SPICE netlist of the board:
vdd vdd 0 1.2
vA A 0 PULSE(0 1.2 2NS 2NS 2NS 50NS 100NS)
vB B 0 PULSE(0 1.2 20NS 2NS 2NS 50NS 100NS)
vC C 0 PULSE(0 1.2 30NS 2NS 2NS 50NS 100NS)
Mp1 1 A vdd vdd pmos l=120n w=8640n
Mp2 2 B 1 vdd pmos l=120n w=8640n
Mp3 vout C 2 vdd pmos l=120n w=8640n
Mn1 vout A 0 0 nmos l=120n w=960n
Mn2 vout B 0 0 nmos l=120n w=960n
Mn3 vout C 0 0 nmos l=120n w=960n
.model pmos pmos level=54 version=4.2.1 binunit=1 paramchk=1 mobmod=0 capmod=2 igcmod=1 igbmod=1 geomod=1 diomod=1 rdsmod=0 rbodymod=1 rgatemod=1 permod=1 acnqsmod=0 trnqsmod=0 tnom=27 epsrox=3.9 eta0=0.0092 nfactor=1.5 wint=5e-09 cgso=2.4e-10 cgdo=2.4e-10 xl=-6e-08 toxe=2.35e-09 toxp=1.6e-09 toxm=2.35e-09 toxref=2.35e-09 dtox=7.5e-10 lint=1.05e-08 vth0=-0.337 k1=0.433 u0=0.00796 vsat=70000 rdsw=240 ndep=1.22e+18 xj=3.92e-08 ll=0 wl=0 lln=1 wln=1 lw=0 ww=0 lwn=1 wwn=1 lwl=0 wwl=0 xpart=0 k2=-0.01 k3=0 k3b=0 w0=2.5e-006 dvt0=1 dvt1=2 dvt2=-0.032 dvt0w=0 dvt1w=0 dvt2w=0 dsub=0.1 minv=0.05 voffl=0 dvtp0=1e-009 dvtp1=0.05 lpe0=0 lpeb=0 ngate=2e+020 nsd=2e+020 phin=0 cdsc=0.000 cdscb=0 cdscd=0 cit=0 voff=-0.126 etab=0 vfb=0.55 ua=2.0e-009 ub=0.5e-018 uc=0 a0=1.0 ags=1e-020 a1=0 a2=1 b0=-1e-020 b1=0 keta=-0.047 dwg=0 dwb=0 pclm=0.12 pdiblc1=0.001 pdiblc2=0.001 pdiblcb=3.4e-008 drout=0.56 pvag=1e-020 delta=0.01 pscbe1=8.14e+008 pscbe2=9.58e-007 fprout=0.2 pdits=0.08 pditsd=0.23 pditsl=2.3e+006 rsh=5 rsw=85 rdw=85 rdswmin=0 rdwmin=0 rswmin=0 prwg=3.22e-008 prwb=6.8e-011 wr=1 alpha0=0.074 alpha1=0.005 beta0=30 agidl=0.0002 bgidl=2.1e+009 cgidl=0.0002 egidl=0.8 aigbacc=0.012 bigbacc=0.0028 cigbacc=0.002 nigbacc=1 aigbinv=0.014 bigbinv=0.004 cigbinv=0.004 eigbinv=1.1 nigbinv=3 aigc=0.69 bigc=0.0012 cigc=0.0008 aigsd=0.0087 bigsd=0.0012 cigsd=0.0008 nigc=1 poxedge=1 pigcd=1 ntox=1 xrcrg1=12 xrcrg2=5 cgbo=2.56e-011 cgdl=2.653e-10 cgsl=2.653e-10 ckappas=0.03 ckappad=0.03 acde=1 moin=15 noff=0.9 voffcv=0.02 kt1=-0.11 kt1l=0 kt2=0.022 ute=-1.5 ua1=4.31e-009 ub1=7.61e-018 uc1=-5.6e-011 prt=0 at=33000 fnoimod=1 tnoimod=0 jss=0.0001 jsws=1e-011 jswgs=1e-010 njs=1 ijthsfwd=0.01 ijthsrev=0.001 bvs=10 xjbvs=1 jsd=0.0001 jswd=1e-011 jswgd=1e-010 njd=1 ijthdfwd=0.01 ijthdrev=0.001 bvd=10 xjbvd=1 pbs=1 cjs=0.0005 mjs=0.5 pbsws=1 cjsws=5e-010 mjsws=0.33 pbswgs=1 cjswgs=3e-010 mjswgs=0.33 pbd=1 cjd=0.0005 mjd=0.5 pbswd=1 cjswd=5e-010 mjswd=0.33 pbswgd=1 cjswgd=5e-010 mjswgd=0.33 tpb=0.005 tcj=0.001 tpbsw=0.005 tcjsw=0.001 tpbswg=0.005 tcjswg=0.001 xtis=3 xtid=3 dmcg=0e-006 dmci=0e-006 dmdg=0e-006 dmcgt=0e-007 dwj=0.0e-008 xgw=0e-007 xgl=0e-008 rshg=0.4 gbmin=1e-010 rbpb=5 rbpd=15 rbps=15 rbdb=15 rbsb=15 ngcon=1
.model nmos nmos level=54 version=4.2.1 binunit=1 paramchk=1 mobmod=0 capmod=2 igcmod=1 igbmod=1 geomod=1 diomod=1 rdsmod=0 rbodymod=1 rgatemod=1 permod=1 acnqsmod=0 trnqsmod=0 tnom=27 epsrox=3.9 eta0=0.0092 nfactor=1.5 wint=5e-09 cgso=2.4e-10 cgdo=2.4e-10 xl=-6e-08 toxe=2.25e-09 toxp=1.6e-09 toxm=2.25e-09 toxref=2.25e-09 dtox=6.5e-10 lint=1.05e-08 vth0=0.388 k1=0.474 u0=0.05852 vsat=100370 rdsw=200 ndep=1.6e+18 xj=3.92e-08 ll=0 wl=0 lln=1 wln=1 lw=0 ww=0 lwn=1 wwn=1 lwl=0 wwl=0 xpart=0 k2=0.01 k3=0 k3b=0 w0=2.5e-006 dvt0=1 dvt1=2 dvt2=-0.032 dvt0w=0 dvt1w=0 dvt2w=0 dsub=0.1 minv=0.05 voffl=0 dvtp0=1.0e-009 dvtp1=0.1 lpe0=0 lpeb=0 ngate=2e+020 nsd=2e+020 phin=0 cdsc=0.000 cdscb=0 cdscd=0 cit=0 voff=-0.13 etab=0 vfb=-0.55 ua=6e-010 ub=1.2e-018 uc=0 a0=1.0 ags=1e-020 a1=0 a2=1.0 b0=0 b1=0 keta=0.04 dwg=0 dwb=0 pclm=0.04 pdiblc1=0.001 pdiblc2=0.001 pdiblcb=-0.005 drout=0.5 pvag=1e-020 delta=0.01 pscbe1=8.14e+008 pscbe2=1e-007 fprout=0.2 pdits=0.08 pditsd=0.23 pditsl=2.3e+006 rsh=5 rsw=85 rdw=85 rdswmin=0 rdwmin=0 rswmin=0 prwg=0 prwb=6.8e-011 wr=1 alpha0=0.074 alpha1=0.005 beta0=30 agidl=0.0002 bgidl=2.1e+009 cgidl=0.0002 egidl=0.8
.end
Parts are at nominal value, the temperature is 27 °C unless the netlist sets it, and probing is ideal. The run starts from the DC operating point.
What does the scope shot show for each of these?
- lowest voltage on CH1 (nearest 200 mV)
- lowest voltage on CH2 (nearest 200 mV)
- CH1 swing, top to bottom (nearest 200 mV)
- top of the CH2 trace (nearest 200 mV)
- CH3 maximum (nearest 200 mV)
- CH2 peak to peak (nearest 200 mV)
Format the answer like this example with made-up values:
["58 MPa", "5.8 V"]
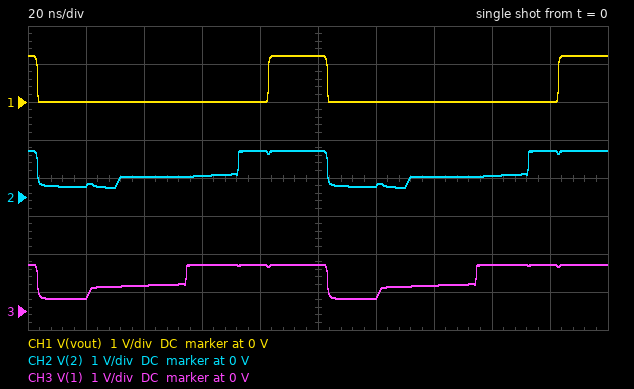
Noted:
["0 V", "200 mV", "1.2 V", "1.2 V", "1.2 V", "1.0 V"]
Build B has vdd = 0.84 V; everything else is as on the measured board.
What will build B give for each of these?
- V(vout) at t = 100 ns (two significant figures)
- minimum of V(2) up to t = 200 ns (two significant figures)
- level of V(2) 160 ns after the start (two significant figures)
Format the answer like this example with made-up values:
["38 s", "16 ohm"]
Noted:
["840 mV", "190 mV", "470 mV"]
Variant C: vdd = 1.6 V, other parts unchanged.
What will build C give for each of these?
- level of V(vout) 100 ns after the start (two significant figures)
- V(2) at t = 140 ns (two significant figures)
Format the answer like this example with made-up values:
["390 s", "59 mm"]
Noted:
["1.6 V", "1.4 V"]
